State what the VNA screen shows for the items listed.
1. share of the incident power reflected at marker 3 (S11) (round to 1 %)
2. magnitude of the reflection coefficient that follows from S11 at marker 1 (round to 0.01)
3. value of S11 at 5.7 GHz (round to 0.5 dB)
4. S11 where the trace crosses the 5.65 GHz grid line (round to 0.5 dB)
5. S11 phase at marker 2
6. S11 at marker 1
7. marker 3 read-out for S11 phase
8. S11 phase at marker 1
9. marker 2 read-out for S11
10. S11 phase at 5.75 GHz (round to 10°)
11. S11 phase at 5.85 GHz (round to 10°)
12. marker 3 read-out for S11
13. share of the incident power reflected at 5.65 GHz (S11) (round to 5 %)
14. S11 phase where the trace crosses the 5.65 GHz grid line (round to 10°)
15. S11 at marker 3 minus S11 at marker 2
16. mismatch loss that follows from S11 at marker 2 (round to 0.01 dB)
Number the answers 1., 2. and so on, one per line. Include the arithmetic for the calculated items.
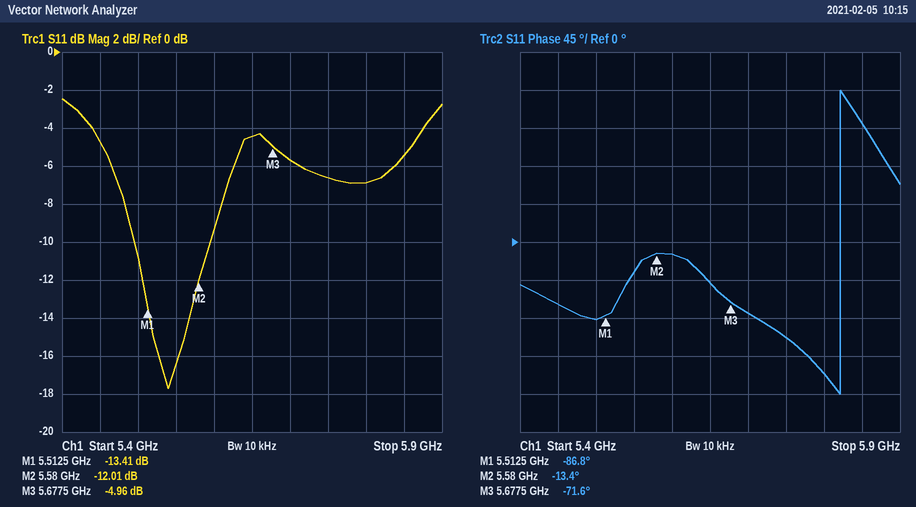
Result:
1. 10^(-4.96/10) ≈ 32 %
2. 10^(-13.41/20) ≈ 0.21
3. -5.5 dB
4. -4.5 dB
5. -13.4°
6. -13.41 dB
7. -71.6°
8. -86.8°
9. -12.01 dB
10. -110°
11. 140°
12. -4.96 dB
13. 10^(-4.5/10) ≈ 35 %
14. -50°
15. -4.96 − (-12.01) = 7.05 dB
16. −10 log10(1 − 10^(-12.01/10)) ≈ 0.28 dB
